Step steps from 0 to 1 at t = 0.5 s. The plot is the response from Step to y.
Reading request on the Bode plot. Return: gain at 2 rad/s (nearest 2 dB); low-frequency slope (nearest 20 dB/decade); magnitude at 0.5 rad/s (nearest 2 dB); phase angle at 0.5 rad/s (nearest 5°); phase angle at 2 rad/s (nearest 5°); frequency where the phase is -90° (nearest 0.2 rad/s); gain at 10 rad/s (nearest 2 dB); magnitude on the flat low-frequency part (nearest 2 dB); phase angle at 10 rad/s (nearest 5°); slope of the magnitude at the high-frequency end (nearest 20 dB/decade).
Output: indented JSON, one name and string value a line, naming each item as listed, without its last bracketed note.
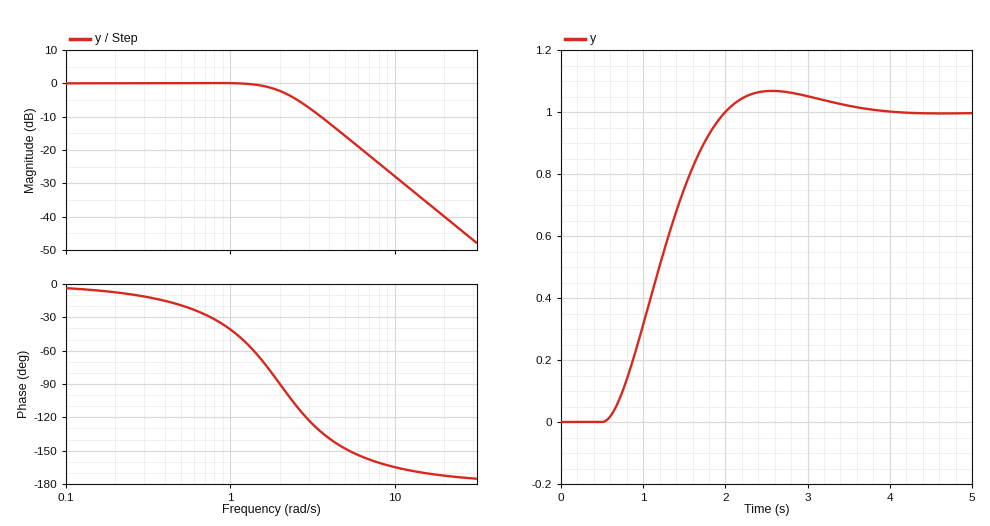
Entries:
{
  "gain at 2 rad/s": "-2 dB",
  "low-frequency slope": "0 dB/decade",
  "magnitude at 0.5 rad/s": "0 dB",
  "phase angle at 0.5 rad/s": "-20°",
  "phase angle at 2 rad/s": "-90°",
  "frequency where the phase is -90°": "2.0 rad/s",
  "gain at 10 rad/s": "-28 dB",
  "magnitude on the flat low-frequency part": "0 dB",
  "phase angle at 10 rad/s": "-165°",
  "slope of the magnitude at the high-frequency end": "-40 dB/decade"
}
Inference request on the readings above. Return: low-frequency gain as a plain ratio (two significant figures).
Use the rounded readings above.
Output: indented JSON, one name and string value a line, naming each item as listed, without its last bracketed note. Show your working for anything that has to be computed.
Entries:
{
  "low-frequency gain as a plain ratio": "10^(0 / 20) = 1.0"
}
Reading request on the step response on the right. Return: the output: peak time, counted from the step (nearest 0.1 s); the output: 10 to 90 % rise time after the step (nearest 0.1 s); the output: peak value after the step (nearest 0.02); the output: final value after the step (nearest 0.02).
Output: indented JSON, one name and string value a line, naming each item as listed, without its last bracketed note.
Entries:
{
  "the output: peak time, counted from the step": "2.1 s",
  "the output: 10 to 90 % rise time after the step": "1.0 s",
  "the output: peak value after the step": "1.06",
  "the output: final value after the step": "1.00"
}
